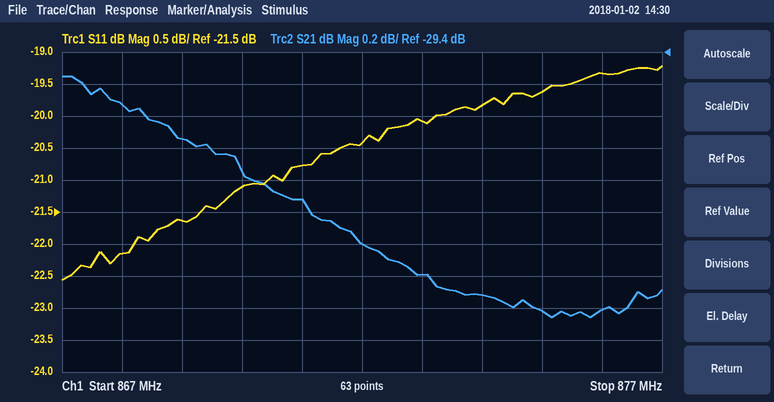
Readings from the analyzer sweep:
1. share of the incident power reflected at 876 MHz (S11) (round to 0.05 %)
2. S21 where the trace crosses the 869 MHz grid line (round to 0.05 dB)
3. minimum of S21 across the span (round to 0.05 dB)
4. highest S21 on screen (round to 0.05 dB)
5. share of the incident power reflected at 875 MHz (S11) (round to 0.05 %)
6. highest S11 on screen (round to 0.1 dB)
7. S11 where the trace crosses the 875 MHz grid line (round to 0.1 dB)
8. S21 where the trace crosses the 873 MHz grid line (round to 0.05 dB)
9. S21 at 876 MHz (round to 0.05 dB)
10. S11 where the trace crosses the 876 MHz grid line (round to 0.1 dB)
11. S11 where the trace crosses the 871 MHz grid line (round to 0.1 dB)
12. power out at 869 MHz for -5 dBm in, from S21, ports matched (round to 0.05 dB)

1.15 %
-29.95 dB
-31.05 dB
-29.55 dB
1.10 %
-19.2 dB
-19.6 dB
-30.80 dB
-31.00 dB
-19.3 dB
-20.8 dB
-34.95 dBm
